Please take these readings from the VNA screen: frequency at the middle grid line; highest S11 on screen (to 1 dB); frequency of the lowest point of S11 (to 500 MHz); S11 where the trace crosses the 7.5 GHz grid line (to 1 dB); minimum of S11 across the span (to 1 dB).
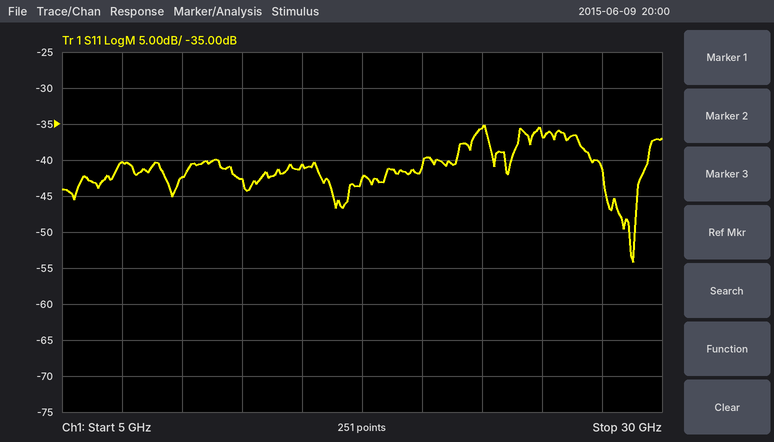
17.5 GHz
-35 dB
29.0 GHz
-40 dB
-54 dB
